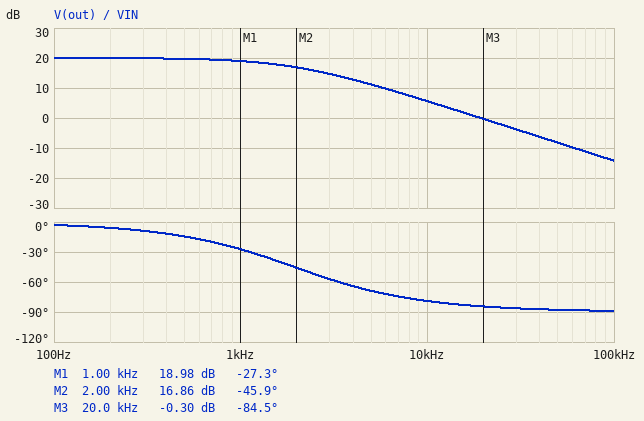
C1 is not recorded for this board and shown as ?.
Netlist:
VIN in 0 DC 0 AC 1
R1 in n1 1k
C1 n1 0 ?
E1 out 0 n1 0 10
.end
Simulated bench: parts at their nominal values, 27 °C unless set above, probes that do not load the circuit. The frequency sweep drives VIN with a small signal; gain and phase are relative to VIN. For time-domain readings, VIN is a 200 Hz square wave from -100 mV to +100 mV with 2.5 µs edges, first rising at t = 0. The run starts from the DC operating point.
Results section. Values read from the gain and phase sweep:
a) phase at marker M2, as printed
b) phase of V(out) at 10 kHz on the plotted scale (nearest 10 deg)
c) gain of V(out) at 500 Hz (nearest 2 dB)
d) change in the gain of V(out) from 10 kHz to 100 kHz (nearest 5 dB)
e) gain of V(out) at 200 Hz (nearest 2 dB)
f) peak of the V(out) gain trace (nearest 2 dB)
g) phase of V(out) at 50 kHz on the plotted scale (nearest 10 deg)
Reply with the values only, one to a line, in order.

-45.9 deg
-80 deg
20 dB
-20 dB
20 dB
20 dB
-90 deg
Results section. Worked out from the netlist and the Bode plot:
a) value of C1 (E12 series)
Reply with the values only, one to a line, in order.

82 nF
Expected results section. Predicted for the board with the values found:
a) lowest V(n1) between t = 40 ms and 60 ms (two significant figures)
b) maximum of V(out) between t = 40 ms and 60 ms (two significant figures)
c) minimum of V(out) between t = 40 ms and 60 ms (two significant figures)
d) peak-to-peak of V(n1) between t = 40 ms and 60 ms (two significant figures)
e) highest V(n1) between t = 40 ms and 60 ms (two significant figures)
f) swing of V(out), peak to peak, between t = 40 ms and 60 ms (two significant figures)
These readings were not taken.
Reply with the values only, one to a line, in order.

-100 mV
1.0 V
-1.0 V
200 mV
100 mV
2.0 V
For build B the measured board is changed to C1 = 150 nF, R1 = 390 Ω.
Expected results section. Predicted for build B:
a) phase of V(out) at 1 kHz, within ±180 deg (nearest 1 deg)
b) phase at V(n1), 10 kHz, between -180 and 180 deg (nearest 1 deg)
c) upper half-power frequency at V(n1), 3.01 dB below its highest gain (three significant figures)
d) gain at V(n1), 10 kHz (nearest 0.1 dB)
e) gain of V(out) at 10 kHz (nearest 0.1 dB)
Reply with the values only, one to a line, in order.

-20 deg
-75 deg
2.72 kHz
-11.6 dB
8.4 dB
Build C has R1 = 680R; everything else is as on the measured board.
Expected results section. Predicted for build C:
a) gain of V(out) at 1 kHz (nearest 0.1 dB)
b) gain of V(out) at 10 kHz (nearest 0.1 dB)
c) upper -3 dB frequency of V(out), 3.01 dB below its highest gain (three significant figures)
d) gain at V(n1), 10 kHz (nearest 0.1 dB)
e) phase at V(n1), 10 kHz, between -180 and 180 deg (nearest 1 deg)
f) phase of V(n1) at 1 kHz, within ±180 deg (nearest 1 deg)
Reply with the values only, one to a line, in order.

19.5 dB
8.8 dB
2.85 kHz
-11.2 dB
-74 deg
-19 deg
